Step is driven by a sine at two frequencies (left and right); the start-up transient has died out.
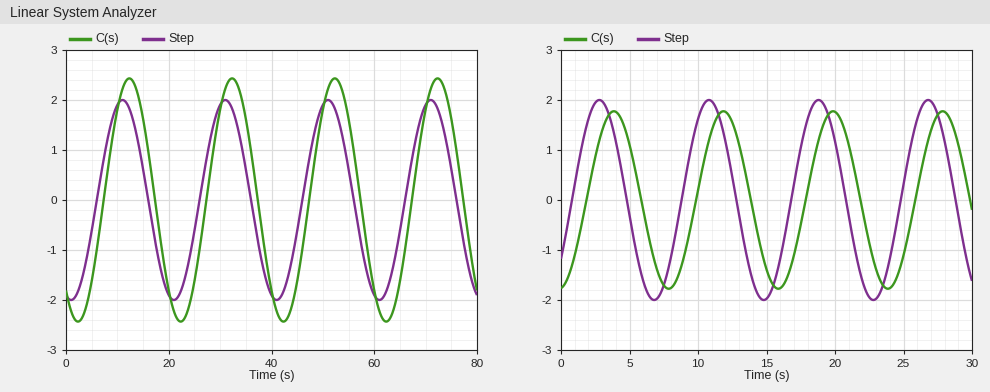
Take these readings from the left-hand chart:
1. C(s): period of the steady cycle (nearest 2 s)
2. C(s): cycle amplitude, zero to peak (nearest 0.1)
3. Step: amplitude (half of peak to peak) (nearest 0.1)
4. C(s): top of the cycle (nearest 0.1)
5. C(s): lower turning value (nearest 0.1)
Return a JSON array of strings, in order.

["20 s", "2.4", "2.0", "2.4", "-2.4"]
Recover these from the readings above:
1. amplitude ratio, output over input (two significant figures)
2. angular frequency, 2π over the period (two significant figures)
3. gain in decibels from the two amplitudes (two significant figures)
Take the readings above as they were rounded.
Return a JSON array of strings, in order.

["1.2", "0.31 rad/s", "1.6 dB"]
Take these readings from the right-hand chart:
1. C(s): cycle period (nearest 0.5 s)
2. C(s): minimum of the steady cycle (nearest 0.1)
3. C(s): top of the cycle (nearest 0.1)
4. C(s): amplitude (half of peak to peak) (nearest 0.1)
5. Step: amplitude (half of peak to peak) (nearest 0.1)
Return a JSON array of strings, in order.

["8.0 s", "-1.8", "1.8", "1.8", "2.0"]
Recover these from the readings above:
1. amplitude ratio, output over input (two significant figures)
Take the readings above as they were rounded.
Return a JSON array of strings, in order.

["0.90"]
